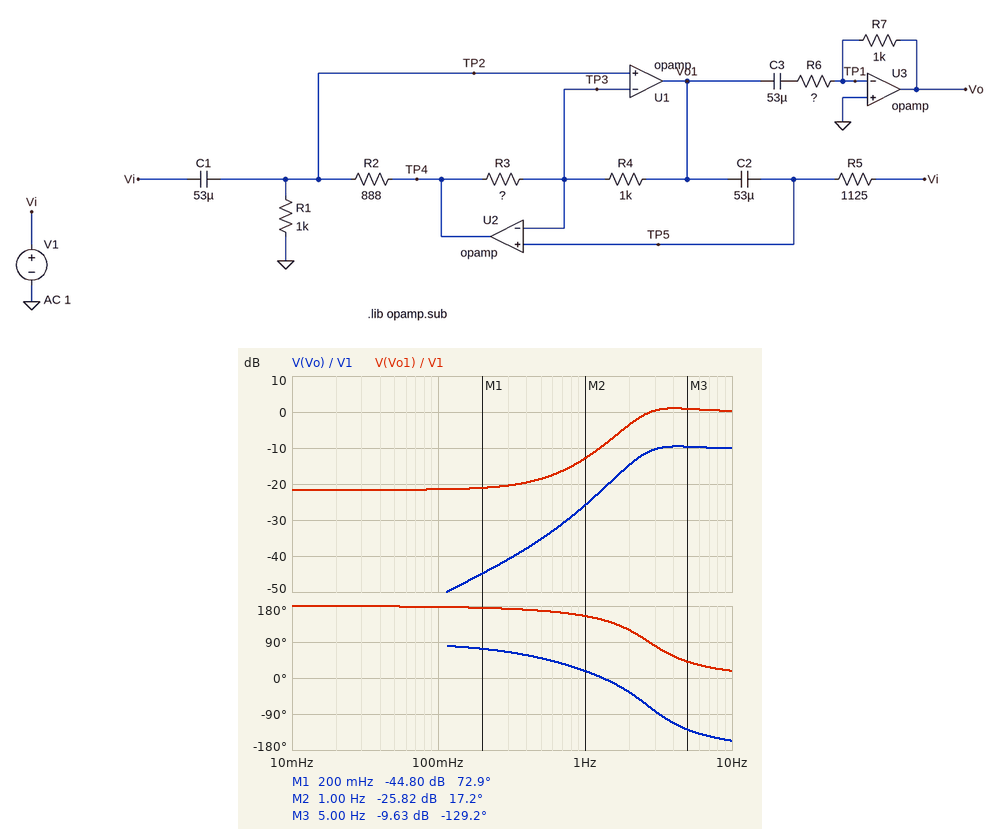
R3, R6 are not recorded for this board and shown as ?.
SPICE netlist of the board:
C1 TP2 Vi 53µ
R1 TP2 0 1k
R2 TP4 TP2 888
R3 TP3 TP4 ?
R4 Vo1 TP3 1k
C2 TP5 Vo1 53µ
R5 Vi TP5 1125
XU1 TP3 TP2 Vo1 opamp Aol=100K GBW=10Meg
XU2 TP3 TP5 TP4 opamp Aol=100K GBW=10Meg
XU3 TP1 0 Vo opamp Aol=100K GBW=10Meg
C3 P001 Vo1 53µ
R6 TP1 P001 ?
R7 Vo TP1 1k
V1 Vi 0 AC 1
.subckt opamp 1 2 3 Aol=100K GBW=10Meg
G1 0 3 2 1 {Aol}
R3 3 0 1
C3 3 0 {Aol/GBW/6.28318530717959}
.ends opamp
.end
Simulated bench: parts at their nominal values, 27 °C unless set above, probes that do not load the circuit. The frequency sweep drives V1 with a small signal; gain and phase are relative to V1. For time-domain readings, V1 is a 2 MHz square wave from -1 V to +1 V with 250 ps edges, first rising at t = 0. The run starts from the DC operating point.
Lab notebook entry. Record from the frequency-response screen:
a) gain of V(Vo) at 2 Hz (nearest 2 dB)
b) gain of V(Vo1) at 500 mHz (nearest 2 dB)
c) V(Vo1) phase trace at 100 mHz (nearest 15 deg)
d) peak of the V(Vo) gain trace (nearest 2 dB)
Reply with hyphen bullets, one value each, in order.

- -14 dB
- -18 dB
- 180 deg
- -10 dB
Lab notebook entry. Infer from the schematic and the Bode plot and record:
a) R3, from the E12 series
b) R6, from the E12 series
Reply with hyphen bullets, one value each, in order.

- 820 Ω
- 3.3 kΩ
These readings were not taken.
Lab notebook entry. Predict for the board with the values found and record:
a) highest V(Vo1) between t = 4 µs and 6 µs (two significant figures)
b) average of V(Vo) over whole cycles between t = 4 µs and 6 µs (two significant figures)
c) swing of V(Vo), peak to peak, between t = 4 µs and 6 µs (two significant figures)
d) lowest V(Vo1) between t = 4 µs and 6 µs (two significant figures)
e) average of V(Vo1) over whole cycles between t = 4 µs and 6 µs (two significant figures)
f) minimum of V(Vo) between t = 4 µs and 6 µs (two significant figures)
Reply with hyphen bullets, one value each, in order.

- 2.5 V
- -300 mV
- 740 mV
- -360 mV
- 1.1 V
- -670 mV
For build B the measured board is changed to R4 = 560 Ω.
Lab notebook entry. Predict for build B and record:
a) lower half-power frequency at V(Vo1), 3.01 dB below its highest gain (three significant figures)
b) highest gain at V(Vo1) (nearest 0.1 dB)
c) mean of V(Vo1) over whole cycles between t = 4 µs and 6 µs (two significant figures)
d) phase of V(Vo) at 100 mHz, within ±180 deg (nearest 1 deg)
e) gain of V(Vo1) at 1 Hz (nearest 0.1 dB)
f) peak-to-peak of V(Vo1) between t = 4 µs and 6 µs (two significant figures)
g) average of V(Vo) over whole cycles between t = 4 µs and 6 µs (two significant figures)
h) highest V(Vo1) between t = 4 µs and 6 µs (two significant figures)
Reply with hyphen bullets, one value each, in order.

- 3.67 Hz
- 0.5 dB
- 610 mV
- -98 deg
- -9.5 dB
- 2.7 V
- -300 mV
- 2.0 V
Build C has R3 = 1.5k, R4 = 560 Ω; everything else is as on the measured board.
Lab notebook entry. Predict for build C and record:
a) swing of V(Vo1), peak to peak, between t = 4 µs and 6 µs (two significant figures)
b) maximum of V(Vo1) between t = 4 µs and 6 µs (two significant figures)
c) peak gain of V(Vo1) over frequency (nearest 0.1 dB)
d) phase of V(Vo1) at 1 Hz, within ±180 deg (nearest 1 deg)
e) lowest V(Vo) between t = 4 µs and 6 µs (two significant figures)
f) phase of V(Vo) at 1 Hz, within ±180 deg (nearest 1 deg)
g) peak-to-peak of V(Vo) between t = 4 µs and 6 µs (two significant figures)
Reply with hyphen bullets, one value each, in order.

- 2.6 V
- 1.6 V
- 0.3 dB
- -7 deg
- -660 mV
- -145 deg
- 720 mV
